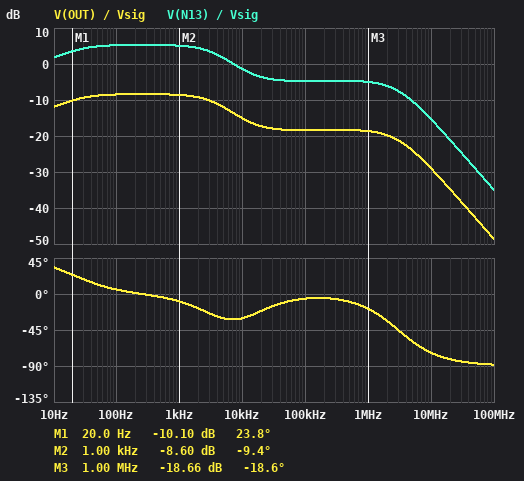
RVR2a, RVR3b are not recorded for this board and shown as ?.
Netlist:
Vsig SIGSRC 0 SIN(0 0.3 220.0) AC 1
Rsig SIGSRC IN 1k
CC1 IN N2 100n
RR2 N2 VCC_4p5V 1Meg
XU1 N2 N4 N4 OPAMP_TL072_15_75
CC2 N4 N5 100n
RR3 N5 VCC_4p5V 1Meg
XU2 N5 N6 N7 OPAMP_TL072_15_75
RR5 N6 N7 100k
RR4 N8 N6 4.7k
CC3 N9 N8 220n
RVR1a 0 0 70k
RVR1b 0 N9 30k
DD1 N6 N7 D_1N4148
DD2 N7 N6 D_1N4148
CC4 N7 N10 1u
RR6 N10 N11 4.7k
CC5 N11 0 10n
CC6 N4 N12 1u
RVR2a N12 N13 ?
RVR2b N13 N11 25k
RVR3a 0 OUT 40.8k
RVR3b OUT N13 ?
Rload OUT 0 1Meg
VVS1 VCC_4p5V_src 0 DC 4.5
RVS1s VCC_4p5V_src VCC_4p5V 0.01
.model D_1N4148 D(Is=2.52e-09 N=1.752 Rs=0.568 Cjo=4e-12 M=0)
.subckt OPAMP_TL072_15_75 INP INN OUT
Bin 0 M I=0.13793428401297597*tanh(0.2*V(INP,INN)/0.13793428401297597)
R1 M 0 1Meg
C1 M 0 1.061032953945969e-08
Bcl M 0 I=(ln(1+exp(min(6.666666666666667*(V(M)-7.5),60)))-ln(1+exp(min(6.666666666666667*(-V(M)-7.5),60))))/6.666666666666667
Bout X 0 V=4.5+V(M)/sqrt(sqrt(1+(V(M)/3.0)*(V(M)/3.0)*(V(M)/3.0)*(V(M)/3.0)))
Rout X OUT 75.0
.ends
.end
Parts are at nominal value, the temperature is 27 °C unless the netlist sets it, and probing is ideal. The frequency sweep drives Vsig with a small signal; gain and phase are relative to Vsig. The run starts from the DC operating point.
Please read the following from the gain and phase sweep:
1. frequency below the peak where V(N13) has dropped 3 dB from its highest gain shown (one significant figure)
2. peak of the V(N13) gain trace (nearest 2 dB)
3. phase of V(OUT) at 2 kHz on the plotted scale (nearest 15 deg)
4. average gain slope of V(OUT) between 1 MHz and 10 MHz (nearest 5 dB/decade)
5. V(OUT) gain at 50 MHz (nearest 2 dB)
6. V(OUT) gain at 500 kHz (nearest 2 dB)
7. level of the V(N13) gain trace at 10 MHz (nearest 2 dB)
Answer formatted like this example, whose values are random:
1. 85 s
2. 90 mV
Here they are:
1. 10 Hz
2. 6 dB
3. -15 deg
4. -10 dB/decade
5. -42 dB
6. -18 dB
7. -16 dB
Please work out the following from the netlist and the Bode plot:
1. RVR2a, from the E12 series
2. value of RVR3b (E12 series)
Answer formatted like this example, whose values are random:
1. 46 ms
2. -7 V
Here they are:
1. 15 kΩ
2. 150 kΩ
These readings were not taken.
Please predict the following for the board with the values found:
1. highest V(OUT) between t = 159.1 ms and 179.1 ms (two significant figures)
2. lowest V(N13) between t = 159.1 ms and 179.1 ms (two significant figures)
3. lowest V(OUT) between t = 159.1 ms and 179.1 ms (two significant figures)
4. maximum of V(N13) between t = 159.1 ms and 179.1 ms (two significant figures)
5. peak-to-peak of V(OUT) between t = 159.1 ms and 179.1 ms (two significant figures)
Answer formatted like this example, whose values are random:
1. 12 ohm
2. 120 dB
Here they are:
1. 81 mV
2. -390 mV
3. -81 mV
4. 390 mV
5. 160 mV
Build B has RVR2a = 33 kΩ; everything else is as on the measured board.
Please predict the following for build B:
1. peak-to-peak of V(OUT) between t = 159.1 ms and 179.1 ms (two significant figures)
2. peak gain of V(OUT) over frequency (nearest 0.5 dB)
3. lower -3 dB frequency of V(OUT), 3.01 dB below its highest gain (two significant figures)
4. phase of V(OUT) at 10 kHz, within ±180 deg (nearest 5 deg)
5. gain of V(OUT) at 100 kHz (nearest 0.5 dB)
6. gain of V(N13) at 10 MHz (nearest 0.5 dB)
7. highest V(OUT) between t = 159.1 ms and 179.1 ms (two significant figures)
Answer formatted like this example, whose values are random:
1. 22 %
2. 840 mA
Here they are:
1. 180 mV
2. -6.5 dB
3. 18 Hz
4. -45 deg
5. -22.0 dB
6. -19.0 dB
7. 91 mV
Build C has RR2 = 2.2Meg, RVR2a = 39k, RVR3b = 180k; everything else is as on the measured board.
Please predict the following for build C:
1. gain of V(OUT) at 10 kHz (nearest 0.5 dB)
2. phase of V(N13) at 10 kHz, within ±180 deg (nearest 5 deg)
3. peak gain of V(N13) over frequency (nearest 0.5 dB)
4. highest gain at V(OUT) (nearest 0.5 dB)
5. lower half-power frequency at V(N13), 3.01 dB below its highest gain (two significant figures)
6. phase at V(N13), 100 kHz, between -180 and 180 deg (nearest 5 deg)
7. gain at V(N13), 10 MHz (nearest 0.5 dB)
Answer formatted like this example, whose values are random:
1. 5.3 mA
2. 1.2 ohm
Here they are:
1. -16.0 dB
2. -50 deg
3. 7.5 dB
4. -7.5 dB
5. 18 Hz
6. -10 deg
7. -19.5 dB
